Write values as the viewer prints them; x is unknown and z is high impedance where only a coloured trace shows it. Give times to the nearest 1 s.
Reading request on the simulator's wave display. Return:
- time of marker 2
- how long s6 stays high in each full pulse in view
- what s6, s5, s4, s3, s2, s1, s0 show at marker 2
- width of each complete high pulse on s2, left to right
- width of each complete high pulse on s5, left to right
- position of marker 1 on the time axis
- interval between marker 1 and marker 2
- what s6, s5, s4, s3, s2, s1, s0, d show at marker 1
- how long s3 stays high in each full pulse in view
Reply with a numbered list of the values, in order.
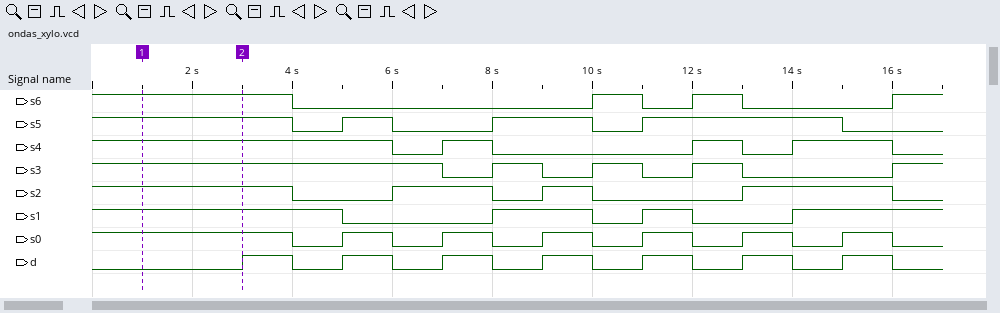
1. 3 s
2. 1 s, 1 s
3. s6=1, s5=1, s4=1, s3=1, s2=1, s1=1, s0=1
4. 2 s, 1 s, 3 s
5. 1 s, 2 s, 4 s
6. 1 s
7. 2 s
8. s6=1, s5=1, s4=1, s3=1, s2=1, s1=1, s0=1, d=0
9. 1 s, 1 s, 1 s
